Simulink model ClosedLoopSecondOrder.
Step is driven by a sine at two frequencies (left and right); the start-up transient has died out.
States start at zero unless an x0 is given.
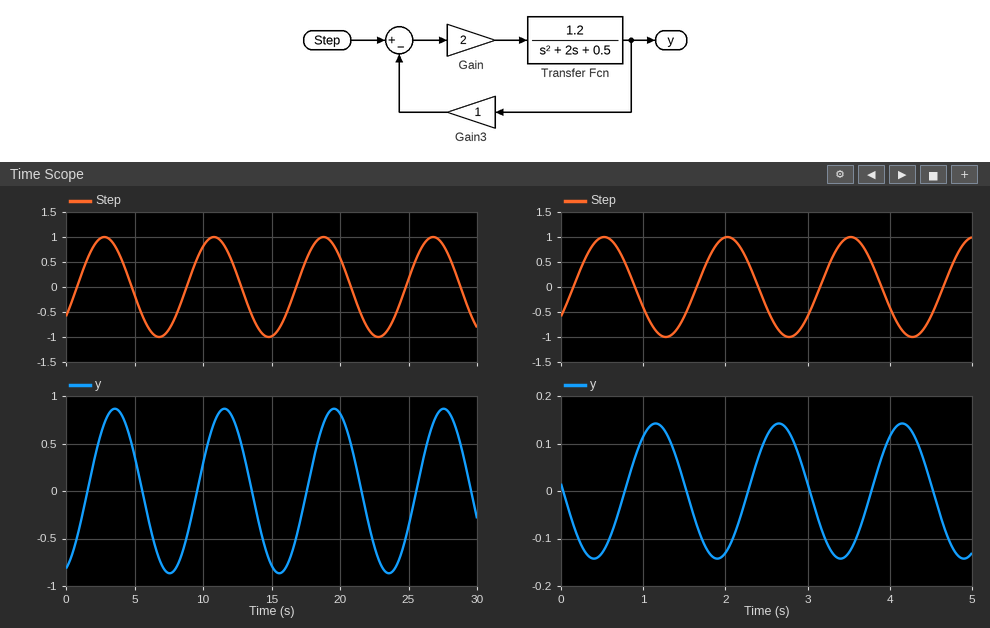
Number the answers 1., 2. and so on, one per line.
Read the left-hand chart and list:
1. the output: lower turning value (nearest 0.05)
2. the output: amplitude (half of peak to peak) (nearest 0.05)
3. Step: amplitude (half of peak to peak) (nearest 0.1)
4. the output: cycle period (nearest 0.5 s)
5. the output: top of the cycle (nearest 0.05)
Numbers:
1. -0.85
2. 0.85
3. 1.0
4. 8.0 s
5. 0.85
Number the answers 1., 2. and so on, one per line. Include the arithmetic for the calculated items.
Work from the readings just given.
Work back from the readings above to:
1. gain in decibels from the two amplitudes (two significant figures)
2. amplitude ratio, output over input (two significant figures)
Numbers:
1. 20 log10(0.85 / 1) = -1.4 dB
2. 0.85 / 1 = 0.85
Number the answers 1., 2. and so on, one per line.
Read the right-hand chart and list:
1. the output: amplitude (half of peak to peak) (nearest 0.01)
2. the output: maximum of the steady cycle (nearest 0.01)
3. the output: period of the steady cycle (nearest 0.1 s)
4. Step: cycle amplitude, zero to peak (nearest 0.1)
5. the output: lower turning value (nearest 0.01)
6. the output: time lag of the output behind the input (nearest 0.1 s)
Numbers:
1. 0.14
2. 0.14
3. 1.5 s
4. 1.0
5. -0.14
6. 0.6 s
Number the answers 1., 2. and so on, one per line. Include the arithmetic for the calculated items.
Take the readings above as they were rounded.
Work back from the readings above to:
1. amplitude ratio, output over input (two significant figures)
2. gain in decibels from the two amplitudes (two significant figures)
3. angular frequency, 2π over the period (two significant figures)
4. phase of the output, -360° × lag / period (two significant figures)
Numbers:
1. 0.14 / 1 = 0.14
2. 20 log10(0.14 / 1) = -17 dB
3. 2π / 1.5 = 4.2 rad/s
4. -360 × 0.6 / 1.5 = -140°
